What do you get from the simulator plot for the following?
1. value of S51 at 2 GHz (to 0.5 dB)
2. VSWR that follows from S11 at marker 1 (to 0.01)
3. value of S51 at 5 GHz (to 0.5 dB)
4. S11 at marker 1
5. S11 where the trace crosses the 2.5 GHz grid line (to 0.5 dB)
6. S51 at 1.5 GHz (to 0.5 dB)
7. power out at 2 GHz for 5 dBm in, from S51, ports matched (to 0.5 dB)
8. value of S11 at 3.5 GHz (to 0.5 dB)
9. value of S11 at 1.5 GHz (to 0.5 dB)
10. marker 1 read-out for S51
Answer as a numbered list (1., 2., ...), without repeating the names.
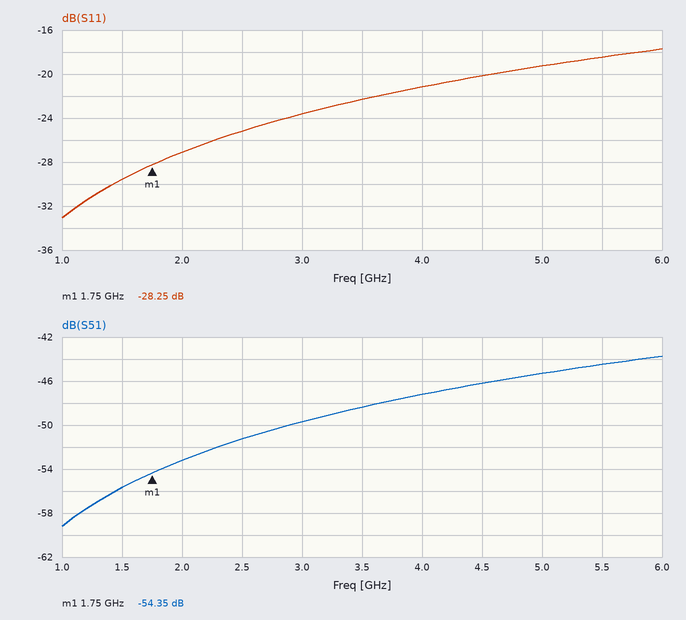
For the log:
1. -53.0 dB
2. 1.08
3. -45.5 dB
4. -28.25 dB
5. -25.0 dB
6. -55.5 dB
7. -48.0 dBm
8. -22.5 dB
9. -29.5 dB
10. -54.35 dB
